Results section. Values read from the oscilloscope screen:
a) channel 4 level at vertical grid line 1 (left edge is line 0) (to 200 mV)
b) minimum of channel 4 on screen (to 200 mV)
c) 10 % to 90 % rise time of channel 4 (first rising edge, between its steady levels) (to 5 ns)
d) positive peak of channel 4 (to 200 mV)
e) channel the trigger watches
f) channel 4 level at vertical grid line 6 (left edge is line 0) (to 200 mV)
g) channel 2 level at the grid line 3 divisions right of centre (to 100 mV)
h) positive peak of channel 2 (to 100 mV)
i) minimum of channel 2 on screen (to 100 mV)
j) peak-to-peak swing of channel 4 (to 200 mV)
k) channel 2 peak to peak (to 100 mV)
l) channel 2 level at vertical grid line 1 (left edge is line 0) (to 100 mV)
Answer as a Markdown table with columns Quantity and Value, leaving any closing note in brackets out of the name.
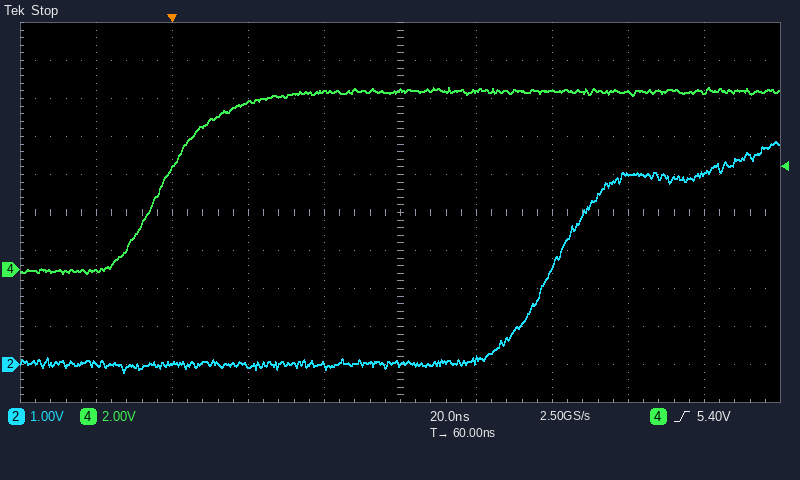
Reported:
| Quantity | Value |
|---|---|
| channel 4 level at vertical grid line 1 (left edge is line 0) | 0.0 V |
| minimum of channel 4 on screen | -200 mV |
| 10 % to 90 % rise time of channel 4 (first rising edge, between its steady levels) | 30 ns |
| positive peak of channel 4 | 9.6 V |
| channel the trigger watches | channel 4 |
| channel 4 level at vertical grid line 6 (left edge is line 0) | 9.4 V |
| channel 2 level at the grid line 3 divisions right of centre | 5.0 V |
| positive peak of channel 2 | 5.9 V |
| minimum of channel 2 on screen | -200 mV |
| peak-to-peak swing of channel 4 | 9.8 V |
| channel 2 peak to peak | 6.1 V |
| channel 2 level at vertical grid line 1 (left edge is line 0) | 0.0 V |
